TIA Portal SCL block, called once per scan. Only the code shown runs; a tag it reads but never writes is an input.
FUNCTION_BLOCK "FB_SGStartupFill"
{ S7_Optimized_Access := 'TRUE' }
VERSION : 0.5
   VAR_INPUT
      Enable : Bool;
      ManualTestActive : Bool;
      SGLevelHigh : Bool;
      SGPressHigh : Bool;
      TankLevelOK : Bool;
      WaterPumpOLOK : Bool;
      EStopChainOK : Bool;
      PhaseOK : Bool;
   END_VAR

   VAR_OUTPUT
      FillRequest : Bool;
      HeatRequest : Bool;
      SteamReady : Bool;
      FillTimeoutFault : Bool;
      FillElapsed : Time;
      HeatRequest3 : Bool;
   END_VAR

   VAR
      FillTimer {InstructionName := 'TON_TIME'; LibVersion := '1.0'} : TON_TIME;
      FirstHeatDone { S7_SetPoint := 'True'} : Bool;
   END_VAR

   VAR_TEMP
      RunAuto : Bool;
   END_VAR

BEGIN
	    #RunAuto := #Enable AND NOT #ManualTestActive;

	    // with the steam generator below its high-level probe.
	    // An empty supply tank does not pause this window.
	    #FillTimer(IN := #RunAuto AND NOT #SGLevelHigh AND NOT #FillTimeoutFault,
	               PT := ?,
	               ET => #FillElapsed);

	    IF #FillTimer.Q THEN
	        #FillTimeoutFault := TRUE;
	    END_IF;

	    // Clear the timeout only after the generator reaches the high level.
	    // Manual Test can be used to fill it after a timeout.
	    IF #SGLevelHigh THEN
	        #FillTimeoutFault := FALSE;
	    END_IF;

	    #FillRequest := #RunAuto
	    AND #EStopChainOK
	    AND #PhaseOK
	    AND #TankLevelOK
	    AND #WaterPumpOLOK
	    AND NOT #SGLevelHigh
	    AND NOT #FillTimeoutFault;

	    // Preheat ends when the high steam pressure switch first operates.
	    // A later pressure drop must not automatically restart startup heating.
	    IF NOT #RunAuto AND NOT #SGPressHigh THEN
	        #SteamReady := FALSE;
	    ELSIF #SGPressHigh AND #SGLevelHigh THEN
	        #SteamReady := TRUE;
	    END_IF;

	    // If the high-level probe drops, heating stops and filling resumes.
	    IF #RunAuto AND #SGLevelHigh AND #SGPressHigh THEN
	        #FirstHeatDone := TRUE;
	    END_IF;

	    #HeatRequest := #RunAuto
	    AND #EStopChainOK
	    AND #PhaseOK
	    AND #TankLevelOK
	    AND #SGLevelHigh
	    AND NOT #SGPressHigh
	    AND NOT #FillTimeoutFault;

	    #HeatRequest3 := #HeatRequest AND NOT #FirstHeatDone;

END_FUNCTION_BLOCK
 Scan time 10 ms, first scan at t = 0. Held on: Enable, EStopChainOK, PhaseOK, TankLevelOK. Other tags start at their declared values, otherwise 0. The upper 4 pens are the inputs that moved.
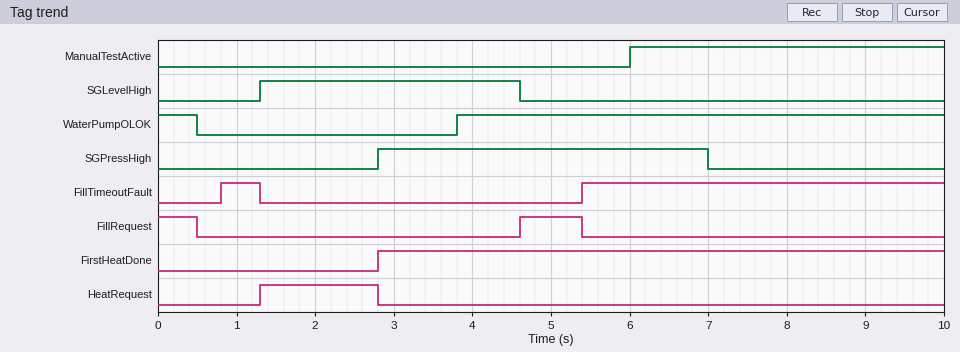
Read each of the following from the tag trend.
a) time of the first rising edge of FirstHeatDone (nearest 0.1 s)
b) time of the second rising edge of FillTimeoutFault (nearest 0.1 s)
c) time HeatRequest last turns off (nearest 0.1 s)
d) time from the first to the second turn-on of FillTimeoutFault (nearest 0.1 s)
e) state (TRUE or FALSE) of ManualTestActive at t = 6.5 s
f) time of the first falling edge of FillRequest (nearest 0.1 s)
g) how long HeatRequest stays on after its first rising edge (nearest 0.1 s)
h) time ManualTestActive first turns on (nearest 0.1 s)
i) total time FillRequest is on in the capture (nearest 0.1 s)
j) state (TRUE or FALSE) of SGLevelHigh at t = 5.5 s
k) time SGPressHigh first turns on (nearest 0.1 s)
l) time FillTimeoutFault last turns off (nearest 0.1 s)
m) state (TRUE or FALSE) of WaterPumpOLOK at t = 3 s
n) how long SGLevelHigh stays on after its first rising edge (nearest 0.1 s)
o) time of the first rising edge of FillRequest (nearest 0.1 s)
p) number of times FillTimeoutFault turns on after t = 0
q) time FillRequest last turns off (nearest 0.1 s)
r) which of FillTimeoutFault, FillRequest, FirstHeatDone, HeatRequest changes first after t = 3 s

2.8 s
5.4 s
2.8 s
4.6 s
TRUE
0.5 s
1.5 s
6.0 s
1.3 s
FALSE
2.8 s
1.3 s
FALSE
3.3 s
4.6 s
2
5.4 s
FillRequest
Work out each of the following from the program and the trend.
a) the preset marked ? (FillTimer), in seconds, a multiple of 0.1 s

0.8 s
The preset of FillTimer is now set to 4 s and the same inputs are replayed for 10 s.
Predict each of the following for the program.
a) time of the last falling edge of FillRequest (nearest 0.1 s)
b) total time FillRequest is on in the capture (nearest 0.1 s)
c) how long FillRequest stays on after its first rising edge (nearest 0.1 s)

6.0 s
1.9 s
1.4 s
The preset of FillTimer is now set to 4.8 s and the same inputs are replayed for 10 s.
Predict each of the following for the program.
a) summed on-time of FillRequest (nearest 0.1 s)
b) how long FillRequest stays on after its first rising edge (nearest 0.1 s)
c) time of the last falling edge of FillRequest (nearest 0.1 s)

1.9 s
1.4 s
6.0 s
